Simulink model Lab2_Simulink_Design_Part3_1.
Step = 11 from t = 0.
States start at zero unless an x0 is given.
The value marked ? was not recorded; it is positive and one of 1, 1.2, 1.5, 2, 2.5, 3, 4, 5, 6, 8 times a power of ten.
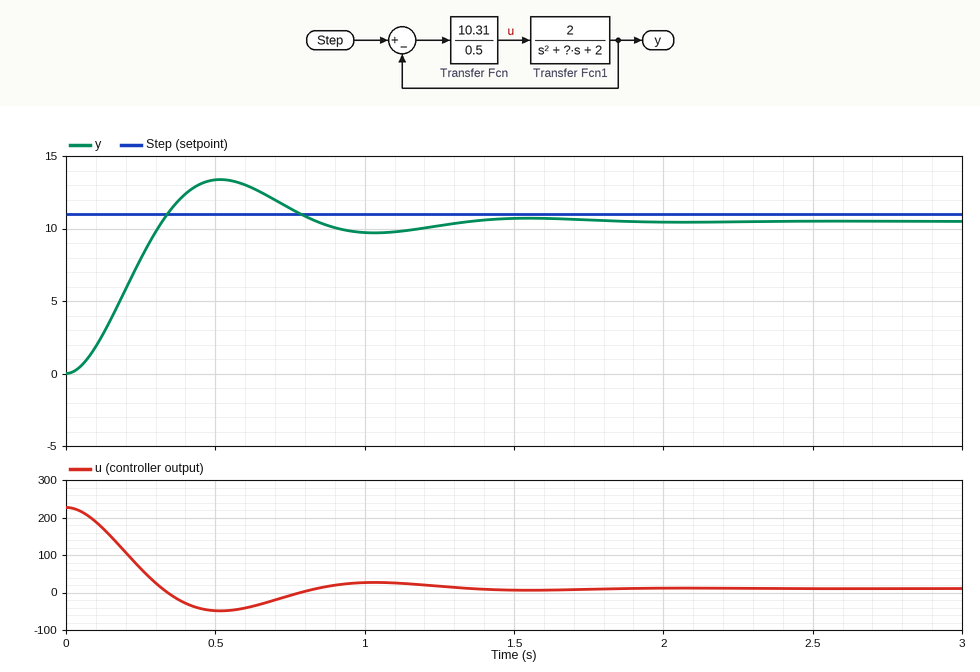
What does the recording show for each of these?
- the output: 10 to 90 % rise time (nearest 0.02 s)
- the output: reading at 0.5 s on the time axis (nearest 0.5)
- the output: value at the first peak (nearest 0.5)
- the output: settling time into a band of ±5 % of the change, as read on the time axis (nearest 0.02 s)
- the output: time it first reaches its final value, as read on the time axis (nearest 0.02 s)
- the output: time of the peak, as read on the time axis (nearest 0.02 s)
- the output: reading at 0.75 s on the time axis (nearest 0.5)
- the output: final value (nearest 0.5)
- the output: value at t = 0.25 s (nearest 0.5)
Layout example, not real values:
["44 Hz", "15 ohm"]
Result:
["0.22 s", "13.5", "13.5", "1.18 s", "0.32 s", "0.52 s", "11.5", "10.5", "8.0"]
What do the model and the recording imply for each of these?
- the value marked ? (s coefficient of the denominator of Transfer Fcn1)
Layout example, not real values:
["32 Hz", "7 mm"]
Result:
["5"]
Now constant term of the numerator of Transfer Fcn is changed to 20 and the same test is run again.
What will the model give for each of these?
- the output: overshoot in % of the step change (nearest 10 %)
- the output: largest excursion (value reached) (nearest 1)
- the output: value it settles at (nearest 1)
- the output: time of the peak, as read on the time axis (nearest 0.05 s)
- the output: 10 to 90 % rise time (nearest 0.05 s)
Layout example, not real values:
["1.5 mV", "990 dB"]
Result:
["40 %", "15", "11", "0.35 s", "0.15 s"]
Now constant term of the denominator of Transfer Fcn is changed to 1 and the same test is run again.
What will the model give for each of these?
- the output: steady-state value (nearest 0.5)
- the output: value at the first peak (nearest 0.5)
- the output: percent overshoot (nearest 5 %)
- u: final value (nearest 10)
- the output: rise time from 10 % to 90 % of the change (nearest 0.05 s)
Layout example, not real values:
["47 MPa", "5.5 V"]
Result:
["10.0", "11.5", "15 %", "10", "0.35 s"]
